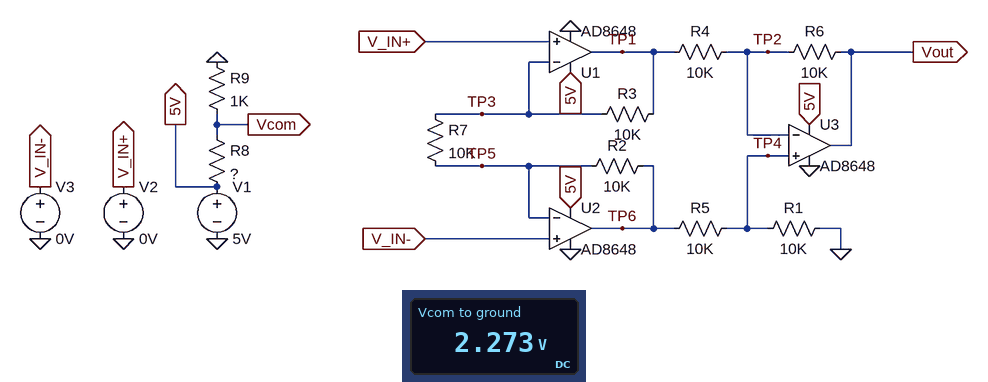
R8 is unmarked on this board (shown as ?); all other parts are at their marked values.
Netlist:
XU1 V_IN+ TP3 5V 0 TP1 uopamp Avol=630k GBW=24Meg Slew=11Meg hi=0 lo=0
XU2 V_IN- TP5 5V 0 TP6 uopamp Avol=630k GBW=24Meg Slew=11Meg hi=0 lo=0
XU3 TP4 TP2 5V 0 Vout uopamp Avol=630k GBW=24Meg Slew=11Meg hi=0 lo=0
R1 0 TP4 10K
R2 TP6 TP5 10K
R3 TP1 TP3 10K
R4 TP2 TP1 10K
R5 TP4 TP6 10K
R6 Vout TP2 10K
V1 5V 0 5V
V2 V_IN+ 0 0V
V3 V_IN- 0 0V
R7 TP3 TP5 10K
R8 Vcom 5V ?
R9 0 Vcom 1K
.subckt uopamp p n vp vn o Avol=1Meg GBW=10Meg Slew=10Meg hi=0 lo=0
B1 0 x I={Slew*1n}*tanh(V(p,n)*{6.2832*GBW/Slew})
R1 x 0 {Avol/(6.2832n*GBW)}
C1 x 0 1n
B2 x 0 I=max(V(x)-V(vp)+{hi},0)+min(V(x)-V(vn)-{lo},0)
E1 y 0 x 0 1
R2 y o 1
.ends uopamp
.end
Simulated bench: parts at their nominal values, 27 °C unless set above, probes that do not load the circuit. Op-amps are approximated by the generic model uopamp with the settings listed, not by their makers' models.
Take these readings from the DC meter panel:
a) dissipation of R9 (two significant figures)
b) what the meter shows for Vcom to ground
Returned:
5.2 mW
2.273 V
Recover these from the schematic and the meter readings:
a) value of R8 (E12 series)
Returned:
1.2 kΩ
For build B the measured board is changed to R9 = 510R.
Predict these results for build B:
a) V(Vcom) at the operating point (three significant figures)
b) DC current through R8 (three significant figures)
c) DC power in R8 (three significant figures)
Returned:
1.49 V
2.92 mA
10.3 mW
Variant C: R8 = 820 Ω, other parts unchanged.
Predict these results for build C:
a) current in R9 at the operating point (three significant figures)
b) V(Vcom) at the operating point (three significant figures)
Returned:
2.75 mA
2.75 V
